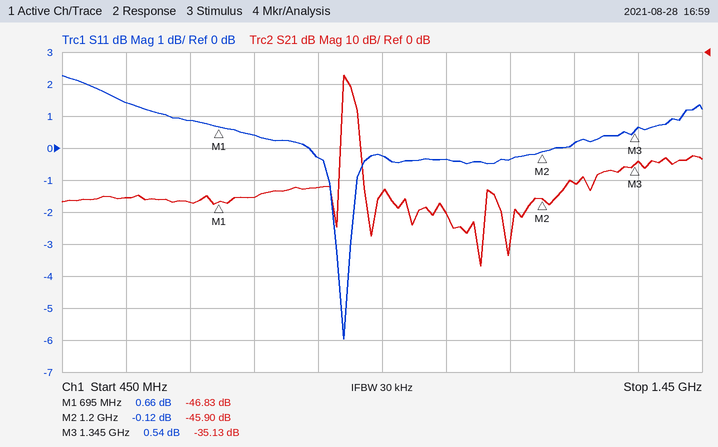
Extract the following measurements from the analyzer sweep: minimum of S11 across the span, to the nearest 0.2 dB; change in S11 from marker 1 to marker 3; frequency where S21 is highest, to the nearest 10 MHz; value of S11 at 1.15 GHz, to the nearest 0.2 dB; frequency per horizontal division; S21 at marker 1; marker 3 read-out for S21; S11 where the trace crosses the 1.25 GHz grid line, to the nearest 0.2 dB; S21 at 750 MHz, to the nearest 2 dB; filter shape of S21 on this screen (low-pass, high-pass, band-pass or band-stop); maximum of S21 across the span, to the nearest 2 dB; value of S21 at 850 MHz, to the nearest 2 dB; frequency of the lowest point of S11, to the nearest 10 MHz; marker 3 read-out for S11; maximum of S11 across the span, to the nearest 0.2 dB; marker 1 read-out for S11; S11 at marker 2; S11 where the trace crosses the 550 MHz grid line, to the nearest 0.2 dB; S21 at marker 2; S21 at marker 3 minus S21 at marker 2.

-6.0 dB
-0.12 dB
890 MHz
-0.4 dB
100 MHz
-46.83 dB
-35.13 dB
0.2 dB
-46 dB
band-pass
-8 dB
-42 dB
890 MHz
0.54 dB
2.2 dB
0.66 dB
-0.12 dB
1.4 dB
-45.90 dB
10.77 dB
